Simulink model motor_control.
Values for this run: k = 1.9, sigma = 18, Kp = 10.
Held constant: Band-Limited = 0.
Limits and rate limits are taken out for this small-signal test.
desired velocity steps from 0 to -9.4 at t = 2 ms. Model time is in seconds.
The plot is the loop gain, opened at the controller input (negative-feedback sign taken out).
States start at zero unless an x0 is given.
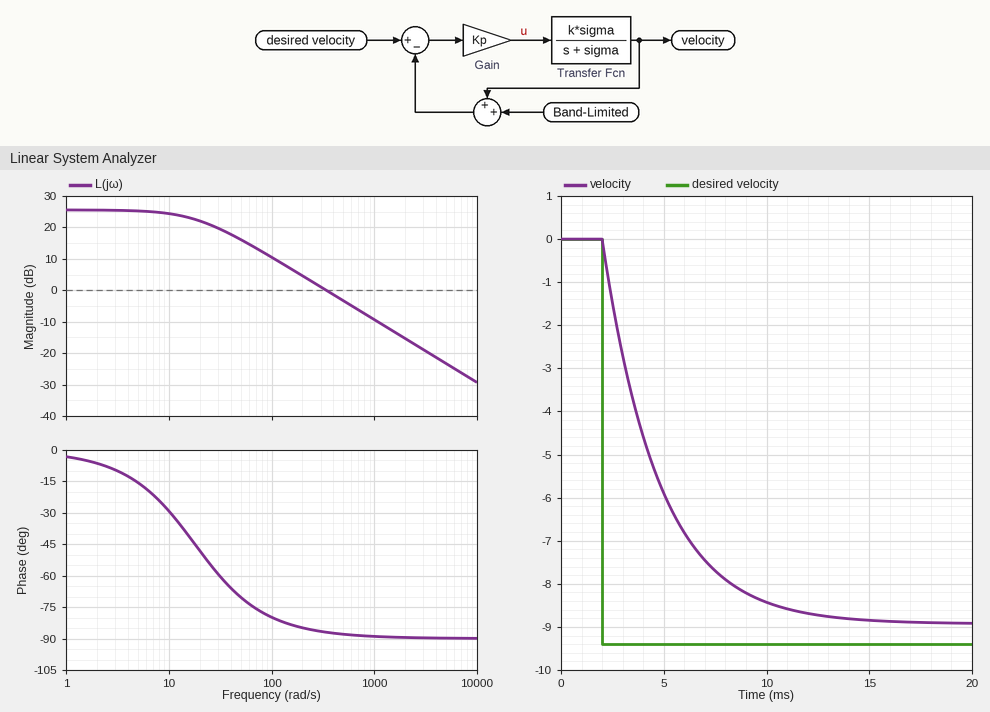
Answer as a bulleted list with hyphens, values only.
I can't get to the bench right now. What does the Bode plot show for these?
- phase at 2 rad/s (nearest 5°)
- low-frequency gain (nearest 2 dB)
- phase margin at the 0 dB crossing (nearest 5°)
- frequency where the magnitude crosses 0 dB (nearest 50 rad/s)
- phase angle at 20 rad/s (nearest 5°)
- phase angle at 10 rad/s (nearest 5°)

- -5°
- 26 dB
- 95°
- 350 rad/s
- -50°
- -30°
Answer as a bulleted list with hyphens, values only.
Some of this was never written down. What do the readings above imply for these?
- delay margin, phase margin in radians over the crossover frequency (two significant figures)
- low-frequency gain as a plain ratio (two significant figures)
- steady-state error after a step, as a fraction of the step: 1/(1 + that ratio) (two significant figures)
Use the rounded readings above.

- 0.0047 s
- 20
- 0.048
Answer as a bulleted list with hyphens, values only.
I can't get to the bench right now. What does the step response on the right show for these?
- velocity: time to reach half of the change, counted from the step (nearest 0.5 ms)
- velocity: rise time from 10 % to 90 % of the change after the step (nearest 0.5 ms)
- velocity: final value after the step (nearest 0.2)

- 2.0 ms
- 6.0 ms
- -9.0
